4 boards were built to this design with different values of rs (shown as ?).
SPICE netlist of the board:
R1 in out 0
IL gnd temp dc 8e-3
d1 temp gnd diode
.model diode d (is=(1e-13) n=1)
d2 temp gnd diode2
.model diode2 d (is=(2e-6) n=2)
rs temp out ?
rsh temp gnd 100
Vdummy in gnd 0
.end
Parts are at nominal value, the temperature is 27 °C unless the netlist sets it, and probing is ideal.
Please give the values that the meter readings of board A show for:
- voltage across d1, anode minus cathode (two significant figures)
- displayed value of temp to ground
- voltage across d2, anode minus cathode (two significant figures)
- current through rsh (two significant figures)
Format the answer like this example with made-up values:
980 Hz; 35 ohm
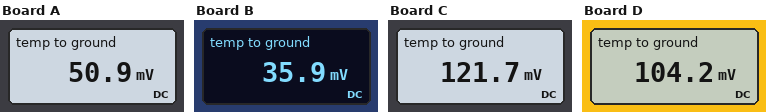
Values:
51 mV; 50.9 mV; 51 mV; 510 µA
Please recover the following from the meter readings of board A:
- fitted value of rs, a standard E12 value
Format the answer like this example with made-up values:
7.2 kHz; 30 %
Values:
6.8 Ω
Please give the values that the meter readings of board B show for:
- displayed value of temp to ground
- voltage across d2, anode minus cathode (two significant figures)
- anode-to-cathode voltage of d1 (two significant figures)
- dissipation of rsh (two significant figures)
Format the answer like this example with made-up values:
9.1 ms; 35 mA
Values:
35.9 mV; 36 mV; 36 mV; 13 µW
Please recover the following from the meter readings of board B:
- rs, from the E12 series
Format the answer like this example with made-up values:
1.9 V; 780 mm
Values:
4.7 Ω
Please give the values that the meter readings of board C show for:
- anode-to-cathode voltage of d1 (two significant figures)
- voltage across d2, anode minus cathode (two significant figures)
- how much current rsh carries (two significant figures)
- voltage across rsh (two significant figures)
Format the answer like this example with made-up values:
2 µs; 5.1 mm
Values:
120 mV; 120 mV; 1.2 mA; 120 mV
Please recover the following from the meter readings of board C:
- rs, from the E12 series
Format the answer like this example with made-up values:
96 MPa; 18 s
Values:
18 Ω
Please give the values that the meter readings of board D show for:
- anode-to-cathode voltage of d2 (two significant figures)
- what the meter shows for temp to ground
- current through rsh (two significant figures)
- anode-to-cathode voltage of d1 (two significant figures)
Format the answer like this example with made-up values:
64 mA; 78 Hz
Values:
100 mV; 104.2 mV; 1.0 mA; 100 mV
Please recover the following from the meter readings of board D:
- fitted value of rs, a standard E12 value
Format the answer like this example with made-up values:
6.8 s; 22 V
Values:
15 Ω
